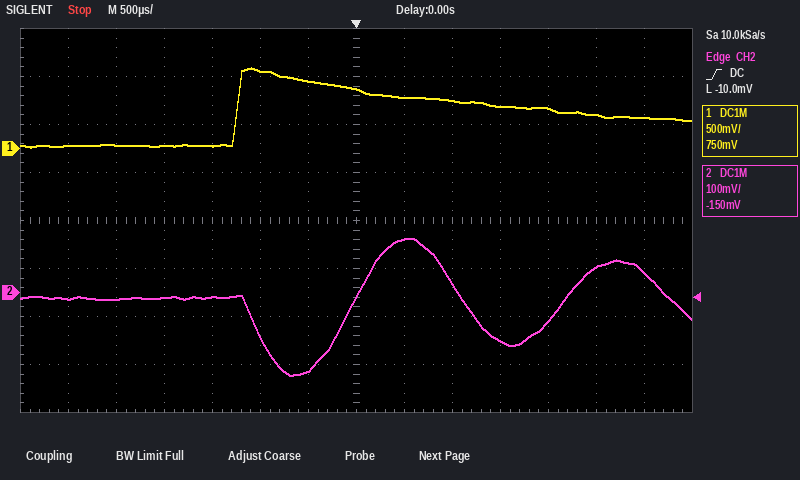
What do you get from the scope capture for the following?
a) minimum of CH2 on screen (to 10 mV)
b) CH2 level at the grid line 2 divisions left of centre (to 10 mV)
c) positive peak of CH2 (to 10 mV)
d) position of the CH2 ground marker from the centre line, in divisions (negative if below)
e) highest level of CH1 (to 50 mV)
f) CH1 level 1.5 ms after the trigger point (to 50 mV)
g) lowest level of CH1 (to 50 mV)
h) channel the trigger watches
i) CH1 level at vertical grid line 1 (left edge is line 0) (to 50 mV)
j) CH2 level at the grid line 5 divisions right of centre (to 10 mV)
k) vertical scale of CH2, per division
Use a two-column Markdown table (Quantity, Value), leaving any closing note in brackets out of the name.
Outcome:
| Quantity | Value |
|---|---|
| minimum of CH2 on screen | -170 mV |
| CH2 level at the grid line 2 divisions left of centre | -90 mV |
| positive peak of CH2 | 110 mV |
| position of the CH2 ground marker from the centre line, in divisions | -1.5 div |
| highest level of CH1 | 850 mV |
| CH1 level 1.5 ms after the trigger point | 450 mV |
| lowest level of CH1 | 0 mV |
| channel the trigger watches | CH2 |
| CH1 level at vertical grid line 1 (left edge is line 0) | 50 mV |
| CH2 level at the grid line 5 divisions right of centre | 50 mV |
| vertical scale of CH2, per division | 100 mV |
